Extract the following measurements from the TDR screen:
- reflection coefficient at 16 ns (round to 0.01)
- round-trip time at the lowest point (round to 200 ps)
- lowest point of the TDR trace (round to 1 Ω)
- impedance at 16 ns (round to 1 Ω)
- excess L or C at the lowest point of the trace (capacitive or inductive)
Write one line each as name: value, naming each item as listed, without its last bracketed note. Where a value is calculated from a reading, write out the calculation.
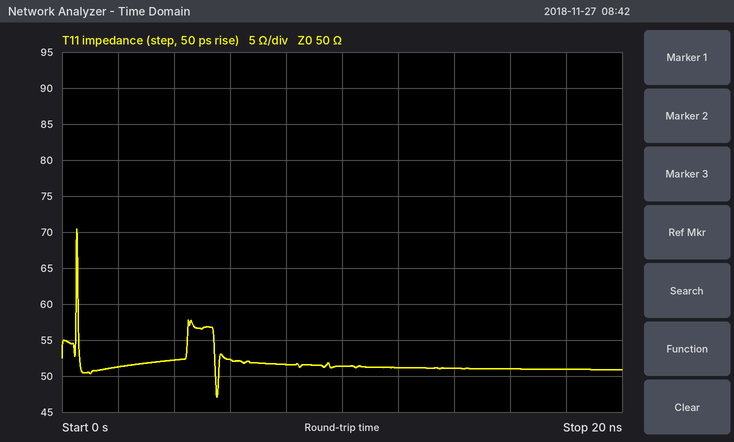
reflection coefficient at 16 ns: (51 − 50)/(51 + 50) ≈ +0.01
round-trip time at the lowest point: 5.6 ns
lowest point of the TDR trace: 47 Ω
impedance at 16 ns: 51 Ω
excess L or C at the lowest point of the trace: capacitive
